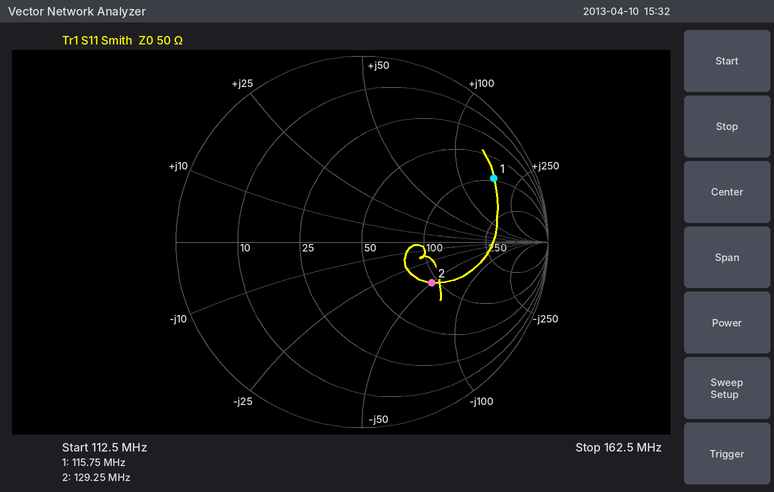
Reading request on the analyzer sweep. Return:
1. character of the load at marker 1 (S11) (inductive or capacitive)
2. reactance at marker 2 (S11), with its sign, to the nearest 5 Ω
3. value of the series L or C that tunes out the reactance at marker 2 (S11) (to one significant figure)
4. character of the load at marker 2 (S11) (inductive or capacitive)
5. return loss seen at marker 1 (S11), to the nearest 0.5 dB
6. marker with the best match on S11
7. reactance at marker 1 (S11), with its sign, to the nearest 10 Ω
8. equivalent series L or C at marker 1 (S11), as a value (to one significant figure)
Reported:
inductive
-50 Ω
60 nH
capacitive
2.0 dB
marker 2
+170 Ω
200 nH
